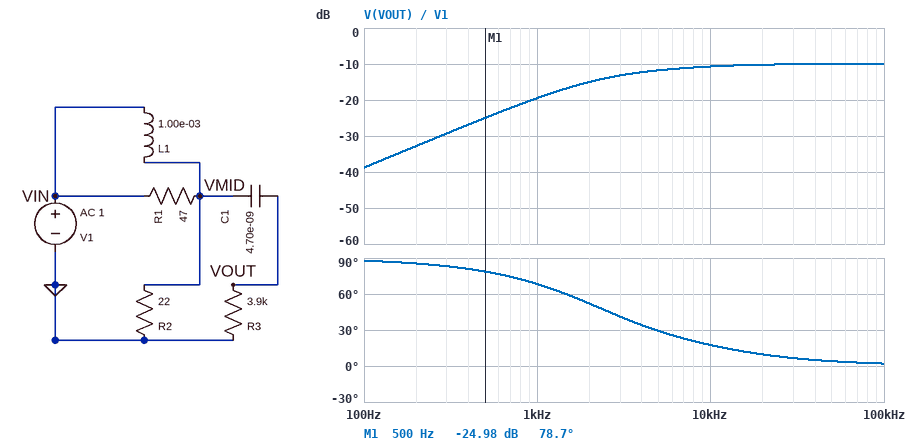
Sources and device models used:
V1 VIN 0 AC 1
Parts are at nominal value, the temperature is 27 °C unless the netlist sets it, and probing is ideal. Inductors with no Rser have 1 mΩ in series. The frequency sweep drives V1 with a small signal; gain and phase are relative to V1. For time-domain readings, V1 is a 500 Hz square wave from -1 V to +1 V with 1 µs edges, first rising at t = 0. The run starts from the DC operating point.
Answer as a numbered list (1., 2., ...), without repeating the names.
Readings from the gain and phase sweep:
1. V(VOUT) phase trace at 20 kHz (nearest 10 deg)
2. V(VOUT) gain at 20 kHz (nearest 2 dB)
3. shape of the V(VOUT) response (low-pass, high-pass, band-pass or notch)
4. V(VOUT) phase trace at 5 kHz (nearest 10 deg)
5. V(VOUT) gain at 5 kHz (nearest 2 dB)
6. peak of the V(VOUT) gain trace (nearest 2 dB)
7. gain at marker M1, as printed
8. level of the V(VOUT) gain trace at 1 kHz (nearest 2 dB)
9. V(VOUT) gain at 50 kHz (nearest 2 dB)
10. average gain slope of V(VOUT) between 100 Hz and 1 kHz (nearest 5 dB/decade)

1. 10 deg
2. -10 dB
3. high-pass
4. 30 deg
5. -12 dB
6. -10 dB
7. -24.98 dB
8. -20 dB
9. -10 dB
10. 20 dB/decade
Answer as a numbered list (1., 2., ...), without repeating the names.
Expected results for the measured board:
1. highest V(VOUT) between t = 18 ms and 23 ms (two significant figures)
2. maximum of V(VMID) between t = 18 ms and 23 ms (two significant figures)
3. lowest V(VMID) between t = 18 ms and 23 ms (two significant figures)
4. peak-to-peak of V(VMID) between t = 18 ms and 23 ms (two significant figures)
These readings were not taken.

1. 630 mV
2. 1.0 V
3. -1.0 V
4. 2.0 V
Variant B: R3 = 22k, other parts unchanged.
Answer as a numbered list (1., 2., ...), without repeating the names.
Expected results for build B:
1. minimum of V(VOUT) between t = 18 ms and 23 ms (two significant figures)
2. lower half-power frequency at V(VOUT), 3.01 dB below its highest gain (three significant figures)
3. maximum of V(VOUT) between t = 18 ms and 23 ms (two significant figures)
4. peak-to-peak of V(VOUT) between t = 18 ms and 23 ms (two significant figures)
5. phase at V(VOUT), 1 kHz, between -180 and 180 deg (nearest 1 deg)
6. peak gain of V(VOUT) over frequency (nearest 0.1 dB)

1. -950 mV
2. 813 Hz
3. 950 mV
4. 1.9 V
5. 42 deg
6. -4.0 dB
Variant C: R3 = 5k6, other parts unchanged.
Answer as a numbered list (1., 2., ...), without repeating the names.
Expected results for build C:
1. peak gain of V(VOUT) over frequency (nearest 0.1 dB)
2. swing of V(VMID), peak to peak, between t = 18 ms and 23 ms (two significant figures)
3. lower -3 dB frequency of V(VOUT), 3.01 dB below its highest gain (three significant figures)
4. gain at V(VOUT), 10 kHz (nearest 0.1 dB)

1. -9.5 dB
2. 2.0 V
3. 1.82 kHz
4. -9.6 dB
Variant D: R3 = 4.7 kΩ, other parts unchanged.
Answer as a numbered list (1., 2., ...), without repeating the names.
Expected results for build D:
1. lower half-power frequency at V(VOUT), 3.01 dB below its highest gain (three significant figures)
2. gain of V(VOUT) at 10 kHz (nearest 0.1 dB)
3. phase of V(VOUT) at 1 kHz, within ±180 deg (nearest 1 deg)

1. 2.22 kHz
2. -10.1 dB
3. 67 deg
